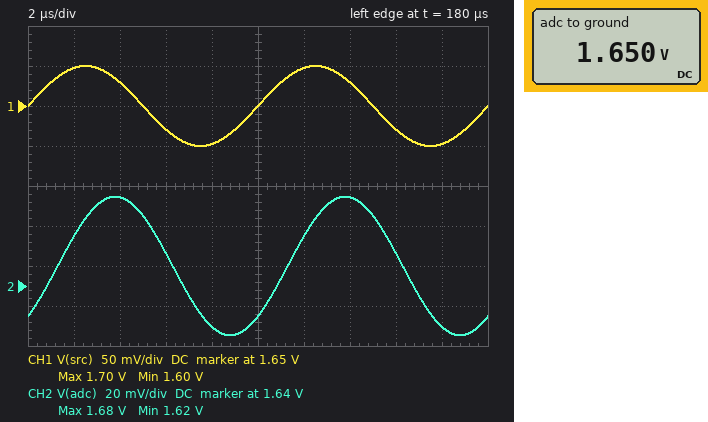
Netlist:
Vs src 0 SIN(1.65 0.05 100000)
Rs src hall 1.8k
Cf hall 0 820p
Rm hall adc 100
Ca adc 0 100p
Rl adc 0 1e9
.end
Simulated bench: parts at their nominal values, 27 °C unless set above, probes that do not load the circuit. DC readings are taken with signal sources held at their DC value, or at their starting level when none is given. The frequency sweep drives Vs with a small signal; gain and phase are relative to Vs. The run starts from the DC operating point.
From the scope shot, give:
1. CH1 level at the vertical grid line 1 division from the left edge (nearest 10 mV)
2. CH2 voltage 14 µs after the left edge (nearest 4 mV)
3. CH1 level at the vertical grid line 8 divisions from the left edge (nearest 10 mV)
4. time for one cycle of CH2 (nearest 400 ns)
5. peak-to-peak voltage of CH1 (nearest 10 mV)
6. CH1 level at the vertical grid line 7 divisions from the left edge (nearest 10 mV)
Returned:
1.70 V
1.684 V
1.62 V
10.0 µs
100 mV
1.68 V
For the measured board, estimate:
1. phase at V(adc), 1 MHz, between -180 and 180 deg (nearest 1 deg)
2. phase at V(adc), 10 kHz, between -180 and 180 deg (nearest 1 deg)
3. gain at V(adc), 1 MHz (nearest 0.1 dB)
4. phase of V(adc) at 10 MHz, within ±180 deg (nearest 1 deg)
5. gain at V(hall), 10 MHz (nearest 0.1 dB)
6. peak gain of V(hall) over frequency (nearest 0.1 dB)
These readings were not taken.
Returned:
-88 deg
-6 deg
-20.4 dB
-119 deg
-40.1 dB
0 dB
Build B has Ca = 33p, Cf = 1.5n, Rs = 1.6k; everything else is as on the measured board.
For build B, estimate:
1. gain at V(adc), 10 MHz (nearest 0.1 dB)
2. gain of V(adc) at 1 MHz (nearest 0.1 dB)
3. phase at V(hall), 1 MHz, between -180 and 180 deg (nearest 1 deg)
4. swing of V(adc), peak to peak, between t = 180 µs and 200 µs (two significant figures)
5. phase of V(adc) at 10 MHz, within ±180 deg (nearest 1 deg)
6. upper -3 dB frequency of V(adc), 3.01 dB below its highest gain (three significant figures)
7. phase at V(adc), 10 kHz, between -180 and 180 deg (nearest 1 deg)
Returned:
-43.9 dB
-23.8 dB
-86 deg
54 mV
-101 deg
64.9 kHz
-9 deg
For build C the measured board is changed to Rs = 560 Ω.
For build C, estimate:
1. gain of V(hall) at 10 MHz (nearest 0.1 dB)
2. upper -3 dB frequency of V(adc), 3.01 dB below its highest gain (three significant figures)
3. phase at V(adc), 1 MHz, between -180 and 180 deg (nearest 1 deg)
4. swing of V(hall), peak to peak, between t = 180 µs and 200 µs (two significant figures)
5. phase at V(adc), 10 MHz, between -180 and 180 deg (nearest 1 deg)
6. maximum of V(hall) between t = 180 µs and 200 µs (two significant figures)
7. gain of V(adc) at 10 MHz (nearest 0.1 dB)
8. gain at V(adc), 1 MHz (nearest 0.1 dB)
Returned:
-30.0 dB
308 kHz
-76 deg
95 mV
-117 deg
1.7 V
-31.4 dB
-10.6 dB
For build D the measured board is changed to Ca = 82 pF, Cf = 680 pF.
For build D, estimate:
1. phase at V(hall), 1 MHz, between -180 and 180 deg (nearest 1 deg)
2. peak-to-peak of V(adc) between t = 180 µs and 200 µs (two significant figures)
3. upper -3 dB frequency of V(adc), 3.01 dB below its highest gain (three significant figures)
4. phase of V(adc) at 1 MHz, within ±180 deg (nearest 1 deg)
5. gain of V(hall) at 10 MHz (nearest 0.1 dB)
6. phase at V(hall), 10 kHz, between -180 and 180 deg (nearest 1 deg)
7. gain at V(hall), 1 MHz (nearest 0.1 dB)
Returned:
-83 deg
76 mV
116 kHz
-86 deg
-38.5 dB
-5 deg
-18.8 dB
